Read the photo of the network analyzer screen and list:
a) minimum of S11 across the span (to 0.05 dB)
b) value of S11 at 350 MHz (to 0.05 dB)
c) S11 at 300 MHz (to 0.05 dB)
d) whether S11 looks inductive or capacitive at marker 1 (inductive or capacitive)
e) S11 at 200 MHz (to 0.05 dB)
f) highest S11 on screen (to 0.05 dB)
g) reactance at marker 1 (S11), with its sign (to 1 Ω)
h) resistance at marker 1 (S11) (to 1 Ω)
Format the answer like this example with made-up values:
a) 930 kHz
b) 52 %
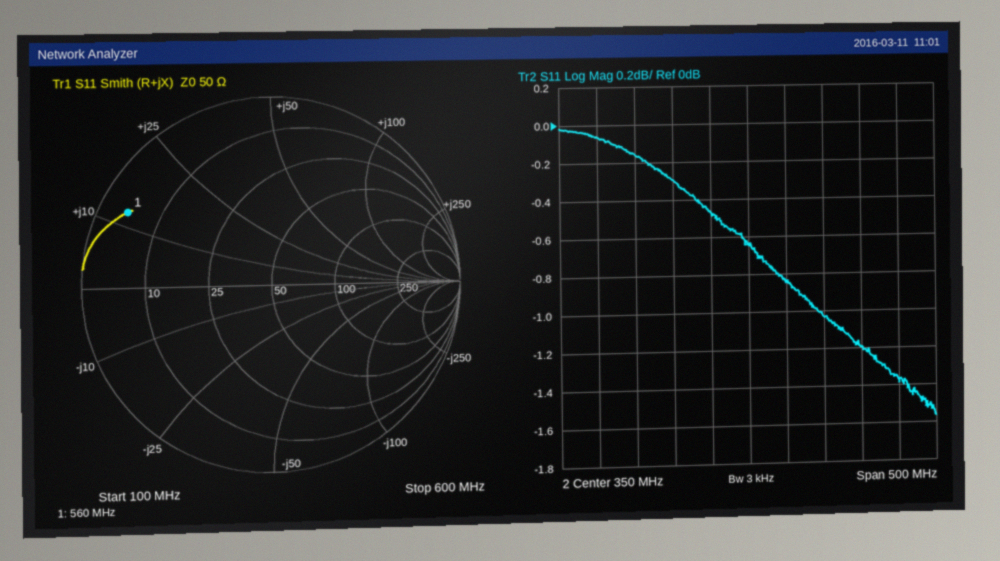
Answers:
a) -1.55 dB
b) -0.65 dB
c) -0.45 dB
d) inductive
e) -0.15 dB
f) 0.00 dB
g) +12 Ω
h) 4 Ω
